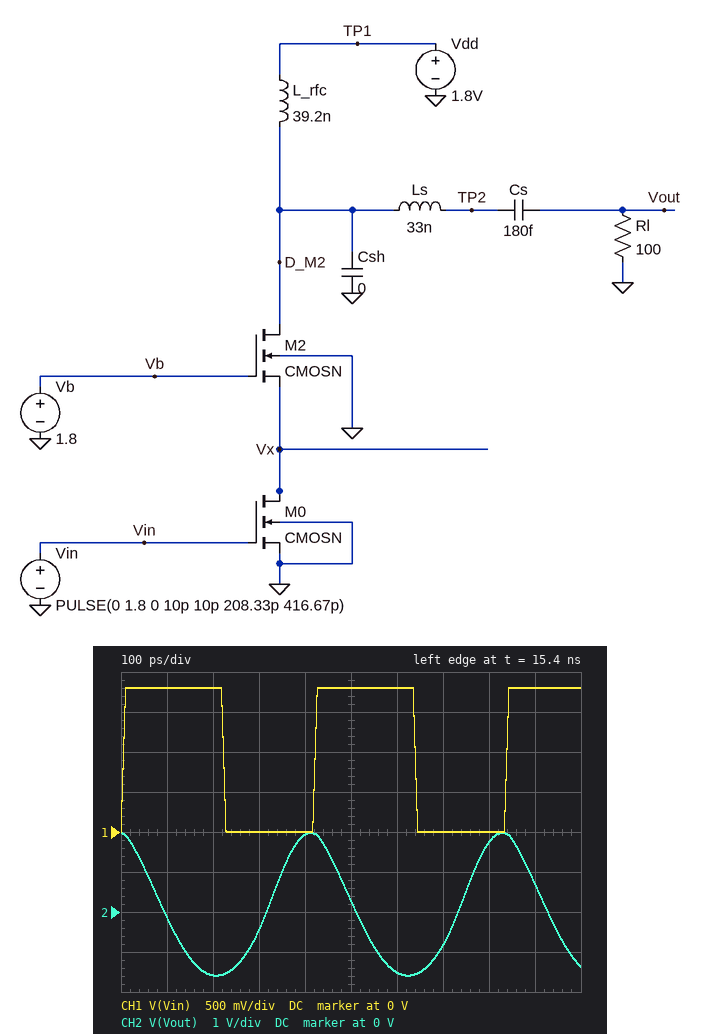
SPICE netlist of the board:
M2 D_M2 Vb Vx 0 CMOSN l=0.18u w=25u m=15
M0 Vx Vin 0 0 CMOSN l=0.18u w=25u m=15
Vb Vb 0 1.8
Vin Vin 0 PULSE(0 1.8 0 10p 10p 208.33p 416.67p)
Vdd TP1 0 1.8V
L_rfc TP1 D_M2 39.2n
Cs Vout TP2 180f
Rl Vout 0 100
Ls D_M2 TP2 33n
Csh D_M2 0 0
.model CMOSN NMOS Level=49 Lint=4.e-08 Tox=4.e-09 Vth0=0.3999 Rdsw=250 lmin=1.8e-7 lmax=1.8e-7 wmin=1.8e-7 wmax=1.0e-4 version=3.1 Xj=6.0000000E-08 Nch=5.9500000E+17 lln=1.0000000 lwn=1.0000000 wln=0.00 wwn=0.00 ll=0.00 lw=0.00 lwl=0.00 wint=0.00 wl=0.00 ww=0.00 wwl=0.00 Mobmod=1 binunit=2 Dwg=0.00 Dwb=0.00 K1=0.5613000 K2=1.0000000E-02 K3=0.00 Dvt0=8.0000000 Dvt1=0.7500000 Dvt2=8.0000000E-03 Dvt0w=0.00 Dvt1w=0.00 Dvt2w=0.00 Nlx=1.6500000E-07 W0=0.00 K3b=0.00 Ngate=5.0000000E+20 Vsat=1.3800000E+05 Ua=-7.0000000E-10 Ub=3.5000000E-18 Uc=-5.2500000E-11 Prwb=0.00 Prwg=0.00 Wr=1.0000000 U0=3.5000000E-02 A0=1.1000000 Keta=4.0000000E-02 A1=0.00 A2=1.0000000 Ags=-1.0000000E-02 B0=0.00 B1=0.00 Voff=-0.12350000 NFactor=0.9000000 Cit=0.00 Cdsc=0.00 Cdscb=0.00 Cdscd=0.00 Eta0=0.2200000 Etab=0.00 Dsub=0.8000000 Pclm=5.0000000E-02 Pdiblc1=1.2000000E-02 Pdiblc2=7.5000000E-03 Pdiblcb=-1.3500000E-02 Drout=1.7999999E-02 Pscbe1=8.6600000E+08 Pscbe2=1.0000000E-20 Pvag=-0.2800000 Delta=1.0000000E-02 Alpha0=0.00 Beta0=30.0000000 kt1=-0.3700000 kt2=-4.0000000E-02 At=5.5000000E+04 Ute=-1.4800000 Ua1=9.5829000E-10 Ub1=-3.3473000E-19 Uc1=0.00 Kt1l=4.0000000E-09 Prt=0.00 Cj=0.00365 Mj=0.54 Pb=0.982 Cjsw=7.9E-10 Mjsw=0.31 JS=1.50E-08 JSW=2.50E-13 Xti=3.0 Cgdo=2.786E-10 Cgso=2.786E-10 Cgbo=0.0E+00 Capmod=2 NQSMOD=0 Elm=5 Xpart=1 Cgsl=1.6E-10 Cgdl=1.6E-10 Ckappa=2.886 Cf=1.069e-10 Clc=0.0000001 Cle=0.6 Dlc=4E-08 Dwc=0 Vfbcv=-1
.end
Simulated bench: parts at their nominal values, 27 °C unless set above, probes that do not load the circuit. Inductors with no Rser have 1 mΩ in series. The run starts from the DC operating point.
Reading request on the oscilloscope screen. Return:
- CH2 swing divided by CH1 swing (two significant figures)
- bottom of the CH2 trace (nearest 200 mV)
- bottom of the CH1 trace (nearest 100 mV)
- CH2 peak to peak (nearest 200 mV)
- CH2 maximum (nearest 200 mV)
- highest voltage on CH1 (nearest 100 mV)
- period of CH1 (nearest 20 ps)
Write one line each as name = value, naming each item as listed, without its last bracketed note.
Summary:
CH2 swing divided by CH1 swing = 2.0
bottom of the CH2 trace = -1.6 V
bottom of the CH1 trace = 0 V
CH2 peak to peak = 3.6 V
CH2 maximum = 2.0 V
highest voltage on CH1 = 1.8 V
period of CH1 = 420 ps
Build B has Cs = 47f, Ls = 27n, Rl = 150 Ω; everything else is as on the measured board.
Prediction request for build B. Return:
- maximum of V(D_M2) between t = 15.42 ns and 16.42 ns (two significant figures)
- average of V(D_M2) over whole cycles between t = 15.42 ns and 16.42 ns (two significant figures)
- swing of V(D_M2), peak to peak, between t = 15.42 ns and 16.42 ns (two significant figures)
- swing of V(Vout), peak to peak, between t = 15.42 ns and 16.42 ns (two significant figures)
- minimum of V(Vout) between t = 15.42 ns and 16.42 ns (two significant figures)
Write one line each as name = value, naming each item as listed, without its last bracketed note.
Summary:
maximum of V(D_M2) between t = 15.42 ns and 16.42 ns = 7.5 V
average of V(D_M2) over whole cycles between t = 15.42 ns and 16.42 ns = 1.8 V
swing of V(D_M2), peak to peak, between t = 15.42 ns and 16.42 ns = 7.7 V
swing of V(Vout), peak to peak, between t = 15.42 ns and 16.42 ns = 3.7 V
minimum of V(Vout) between t = 15.42 ns and 16.42 ns = -2.1 V
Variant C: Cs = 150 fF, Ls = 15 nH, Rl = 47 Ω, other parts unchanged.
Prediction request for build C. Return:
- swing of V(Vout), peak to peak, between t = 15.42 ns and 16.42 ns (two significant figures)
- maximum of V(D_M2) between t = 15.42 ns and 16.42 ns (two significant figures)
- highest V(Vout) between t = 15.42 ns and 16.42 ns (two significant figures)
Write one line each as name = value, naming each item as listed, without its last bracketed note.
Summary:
swing of V(Vout), peak to peak, between t = 15.42 ns and 16.42 ns = 1.9 V
maximum of V(D_M2) between t = 15.42 ns and 16.42 ns = 11 V
highest V(Vout) between t = 15.42 ns and 16.42 ns = 810 mV
